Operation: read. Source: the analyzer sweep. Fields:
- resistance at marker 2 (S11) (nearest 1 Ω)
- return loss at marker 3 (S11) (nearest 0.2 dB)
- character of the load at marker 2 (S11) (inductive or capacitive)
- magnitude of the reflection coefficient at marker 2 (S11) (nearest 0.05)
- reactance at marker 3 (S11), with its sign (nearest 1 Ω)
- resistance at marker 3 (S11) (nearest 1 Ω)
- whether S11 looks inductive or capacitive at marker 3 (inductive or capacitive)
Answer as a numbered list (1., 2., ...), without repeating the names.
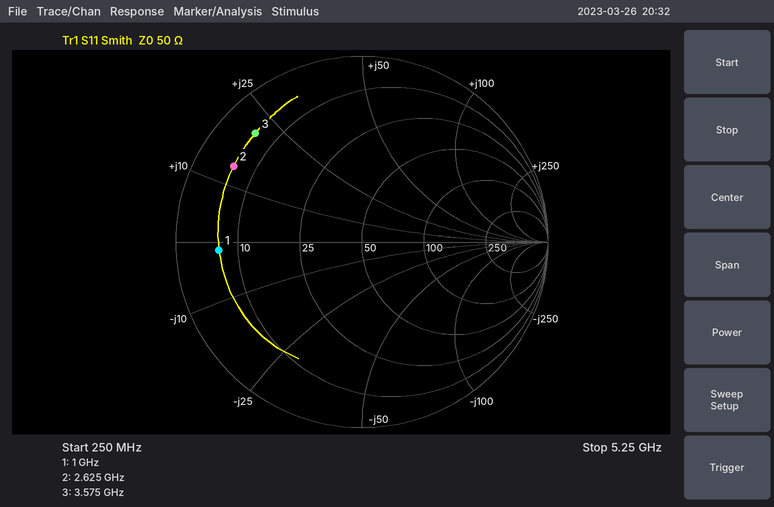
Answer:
1. 6 Ω
2. 1.8 dB
3. inductive
4. 0.80
5. +21 Ω
6. 6 Ω
7. inductive
